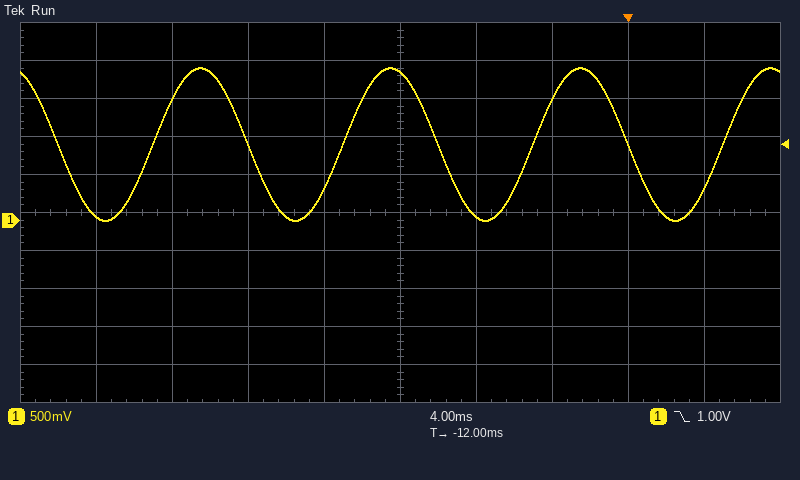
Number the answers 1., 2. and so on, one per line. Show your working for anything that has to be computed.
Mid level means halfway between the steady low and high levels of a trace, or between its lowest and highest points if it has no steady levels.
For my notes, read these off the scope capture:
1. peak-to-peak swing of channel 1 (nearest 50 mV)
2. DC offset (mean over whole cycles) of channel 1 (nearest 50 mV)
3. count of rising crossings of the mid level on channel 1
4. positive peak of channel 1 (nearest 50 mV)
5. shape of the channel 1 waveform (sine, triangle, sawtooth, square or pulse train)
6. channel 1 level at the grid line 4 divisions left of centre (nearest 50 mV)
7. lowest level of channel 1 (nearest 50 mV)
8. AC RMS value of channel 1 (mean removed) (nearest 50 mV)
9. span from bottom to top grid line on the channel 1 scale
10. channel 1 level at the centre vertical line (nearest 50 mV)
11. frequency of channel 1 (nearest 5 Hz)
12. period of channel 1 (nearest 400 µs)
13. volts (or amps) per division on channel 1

1. 2.00 V − (0 mV) = 2.00 V
2. (2.00 V + (0 mV)) / 2 ≈ 1.00 V
3. 4
4. 2.00 V
5. sine
6. 50 mV
7. 0 mV
8. 2.00 V / (2√2) ≈ 707 mV, so 700 mV to the nearest 50 mV
9. 5 V
10. 1.95 V
11. 1 / 10.0 ms ≈ 100 Hz
12. 10.0 ms
13. 500 mV
